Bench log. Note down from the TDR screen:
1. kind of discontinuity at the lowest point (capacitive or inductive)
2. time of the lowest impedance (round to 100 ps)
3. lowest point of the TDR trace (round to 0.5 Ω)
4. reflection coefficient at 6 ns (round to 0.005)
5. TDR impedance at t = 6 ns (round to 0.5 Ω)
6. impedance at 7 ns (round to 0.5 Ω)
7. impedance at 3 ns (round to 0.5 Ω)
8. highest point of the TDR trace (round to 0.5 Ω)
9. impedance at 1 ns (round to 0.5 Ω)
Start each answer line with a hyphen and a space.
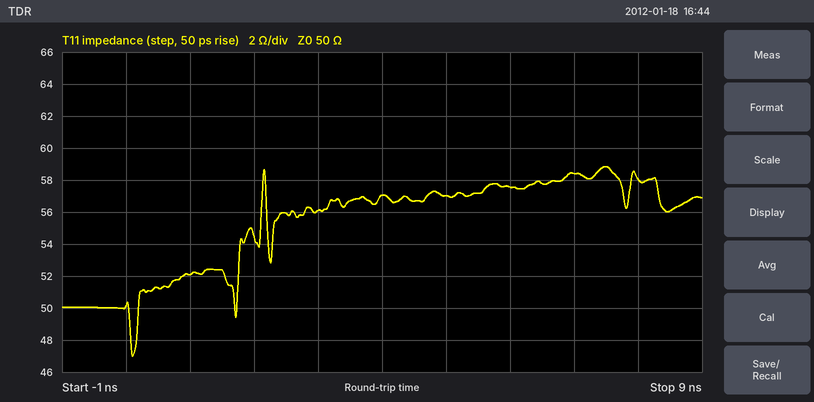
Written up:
- capacitive
- 100 ps
- 47.0 Ω
- +0.070
- 57.5 Ω
- 58.5 Ω
- 56.0 Ω
- 59.0 Ω
- 52.0 Ω
